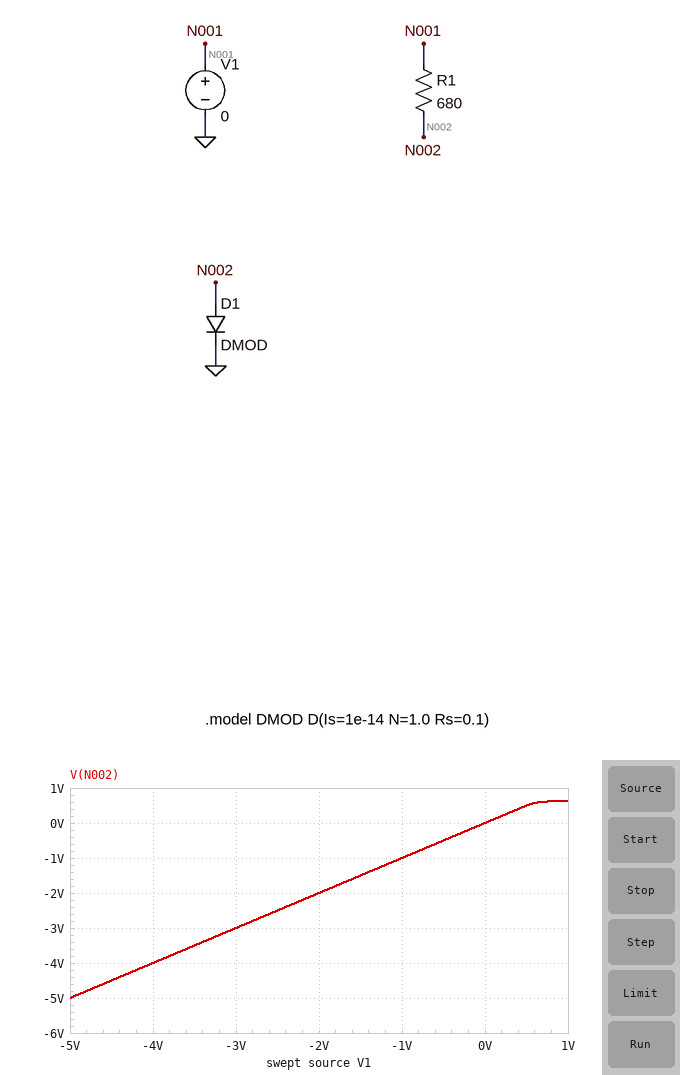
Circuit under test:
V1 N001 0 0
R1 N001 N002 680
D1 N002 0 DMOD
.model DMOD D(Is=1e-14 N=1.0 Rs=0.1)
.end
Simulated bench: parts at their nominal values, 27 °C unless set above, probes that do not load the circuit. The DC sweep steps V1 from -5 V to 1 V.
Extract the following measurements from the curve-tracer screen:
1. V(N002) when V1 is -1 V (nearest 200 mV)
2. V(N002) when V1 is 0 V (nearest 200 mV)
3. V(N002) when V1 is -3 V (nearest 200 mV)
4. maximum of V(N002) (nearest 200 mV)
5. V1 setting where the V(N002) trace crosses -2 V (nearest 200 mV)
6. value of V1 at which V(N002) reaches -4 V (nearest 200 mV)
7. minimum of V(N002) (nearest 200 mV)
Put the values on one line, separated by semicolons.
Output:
-1.0 V; 0 V; -3.0 V; 600 mV; -2.0 V; -4.0 V; -5.0 V
